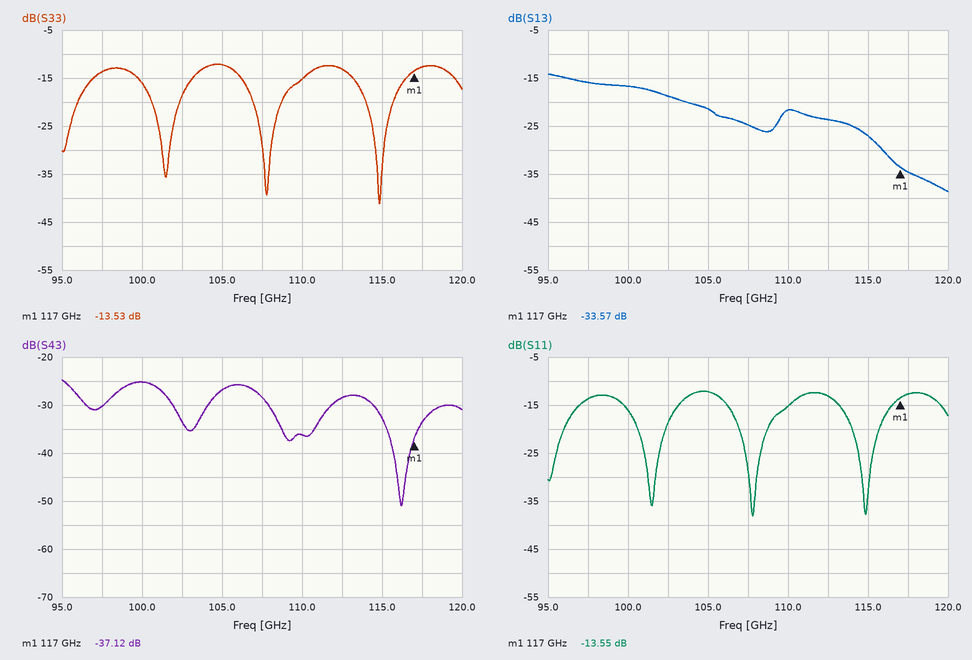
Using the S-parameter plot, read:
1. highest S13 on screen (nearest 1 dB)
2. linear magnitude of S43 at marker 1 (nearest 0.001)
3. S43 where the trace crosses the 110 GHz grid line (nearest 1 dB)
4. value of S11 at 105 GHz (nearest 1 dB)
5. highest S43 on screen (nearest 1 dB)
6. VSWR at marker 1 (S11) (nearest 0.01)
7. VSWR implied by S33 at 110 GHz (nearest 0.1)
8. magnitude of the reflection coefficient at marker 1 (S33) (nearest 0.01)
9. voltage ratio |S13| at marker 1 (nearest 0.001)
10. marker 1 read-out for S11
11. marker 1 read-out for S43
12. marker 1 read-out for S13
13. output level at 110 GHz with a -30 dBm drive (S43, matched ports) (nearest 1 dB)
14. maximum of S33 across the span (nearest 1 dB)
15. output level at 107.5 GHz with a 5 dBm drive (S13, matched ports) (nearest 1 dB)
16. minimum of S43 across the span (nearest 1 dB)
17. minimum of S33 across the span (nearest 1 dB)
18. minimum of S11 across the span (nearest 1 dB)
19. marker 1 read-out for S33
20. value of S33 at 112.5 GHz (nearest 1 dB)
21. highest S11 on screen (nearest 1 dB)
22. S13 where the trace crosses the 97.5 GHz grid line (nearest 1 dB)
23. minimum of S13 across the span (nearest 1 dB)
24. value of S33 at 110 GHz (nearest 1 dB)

-14 dB
0.014
-36 dB
-12 dB
-25 dB
1.53
1.4
0.21
0.021
-13.55 dB
-37.12 dB
-33.57 dB
-66 dBm
-12 dB
-20 dBm
-51 dB
-41 dB
-38 dB
-13.53 dB
-13 dB
-12 dB
-16 dB
-39 dB
-15 dB
